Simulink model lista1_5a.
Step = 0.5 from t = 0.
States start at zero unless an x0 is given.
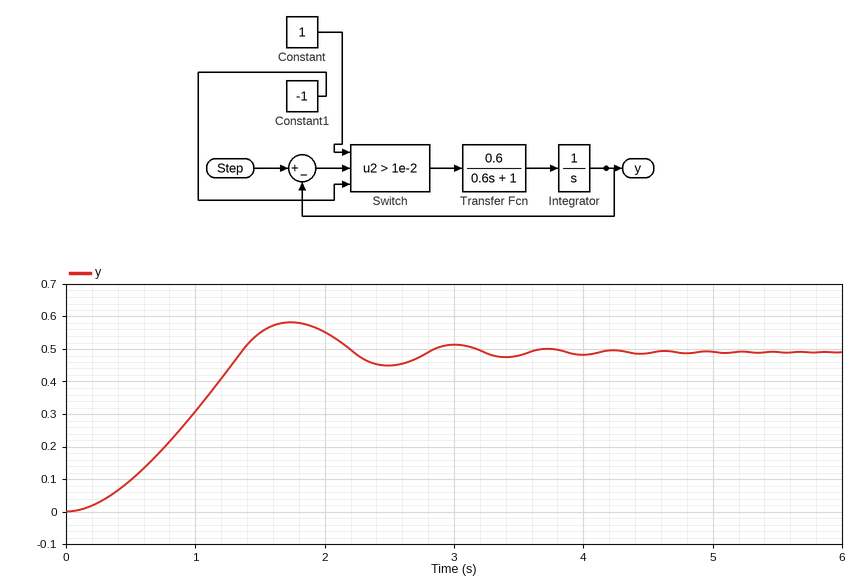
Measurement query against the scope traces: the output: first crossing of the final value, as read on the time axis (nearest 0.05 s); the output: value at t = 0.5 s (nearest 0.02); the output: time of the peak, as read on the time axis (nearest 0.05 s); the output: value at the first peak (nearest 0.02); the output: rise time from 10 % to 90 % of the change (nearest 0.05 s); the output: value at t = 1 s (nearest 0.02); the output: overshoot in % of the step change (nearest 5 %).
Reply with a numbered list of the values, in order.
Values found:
1. 1.35 s
2. 0.10
3. 1.75 s
4. 0.58
5. 0.90 s
6. 0.30
7. 20 %
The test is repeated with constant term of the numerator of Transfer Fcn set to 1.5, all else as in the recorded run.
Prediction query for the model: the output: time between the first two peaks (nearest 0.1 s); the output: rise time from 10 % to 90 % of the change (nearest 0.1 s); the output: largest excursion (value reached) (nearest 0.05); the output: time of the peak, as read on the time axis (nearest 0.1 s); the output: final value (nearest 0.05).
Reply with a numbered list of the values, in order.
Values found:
1. 1.1 s
2. 0.5 s
3. 0.65
4. 1.1 s
5. 0.50
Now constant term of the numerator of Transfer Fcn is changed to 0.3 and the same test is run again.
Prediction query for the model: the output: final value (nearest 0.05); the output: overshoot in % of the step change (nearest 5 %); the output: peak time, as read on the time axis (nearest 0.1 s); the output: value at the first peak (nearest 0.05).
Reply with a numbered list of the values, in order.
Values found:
1. 0.50
2. 10 %
3. 2.6 s
4. 0.55
